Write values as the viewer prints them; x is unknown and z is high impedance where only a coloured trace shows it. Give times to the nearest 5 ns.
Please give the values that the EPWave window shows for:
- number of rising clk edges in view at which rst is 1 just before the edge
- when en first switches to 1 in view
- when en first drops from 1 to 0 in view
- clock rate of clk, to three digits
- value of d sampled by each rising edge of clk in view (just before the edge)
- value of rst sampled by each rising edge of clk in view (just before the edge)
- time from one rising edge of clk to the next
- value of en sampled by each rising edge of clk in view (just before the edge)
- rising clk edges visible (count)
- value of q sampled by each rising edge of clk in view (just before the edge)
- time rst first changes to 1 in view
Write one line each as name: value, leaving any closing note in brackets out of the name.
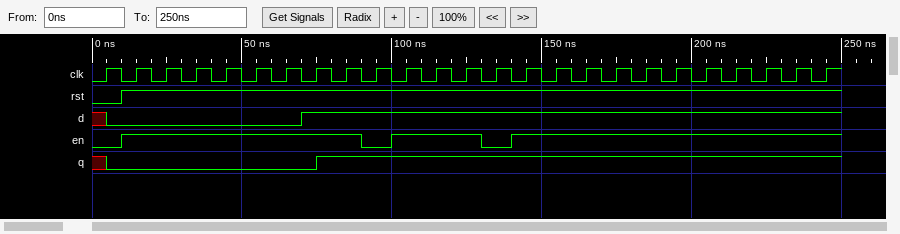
number of rising clk edges in view at which rst is 1 just before the edge: 24
when en first switches to 1 in view: 10 ns
when en first drops from 1 to 0 in view: 90 ns
clock rate of clk, to three digits: 100 MHz
value of d sampled by each rising edge of clk in view: x 0 0 0 0 0 0 1 1 1 1 1 1 1 1 1 1 1 1 1 1 1 1 1 1
value of rst sampled by each rising edge of clk in view: 0 1 1 1 1 1 1 1 1 1 1 1 1 1 1 1 1 1 1 1 1 1 1 1 1
time from one rising edge of clk to the next: 10 ns
value of en sampled by each rising edge of clk in view: 0 1 1 1 1 1 1 1 1 0 1 1 1 0 1 1 1 1 1 1 1 1 1 1 1
rising clk edges visible: 25
value of q sampled by each rising edge of clk in view: x 0 0 0 0 0 0 0 1 1 1 1 1 1 1 1 1 1 1 1 1 1 1 1 1
time rst first changes to 1 in view: 10 ns
